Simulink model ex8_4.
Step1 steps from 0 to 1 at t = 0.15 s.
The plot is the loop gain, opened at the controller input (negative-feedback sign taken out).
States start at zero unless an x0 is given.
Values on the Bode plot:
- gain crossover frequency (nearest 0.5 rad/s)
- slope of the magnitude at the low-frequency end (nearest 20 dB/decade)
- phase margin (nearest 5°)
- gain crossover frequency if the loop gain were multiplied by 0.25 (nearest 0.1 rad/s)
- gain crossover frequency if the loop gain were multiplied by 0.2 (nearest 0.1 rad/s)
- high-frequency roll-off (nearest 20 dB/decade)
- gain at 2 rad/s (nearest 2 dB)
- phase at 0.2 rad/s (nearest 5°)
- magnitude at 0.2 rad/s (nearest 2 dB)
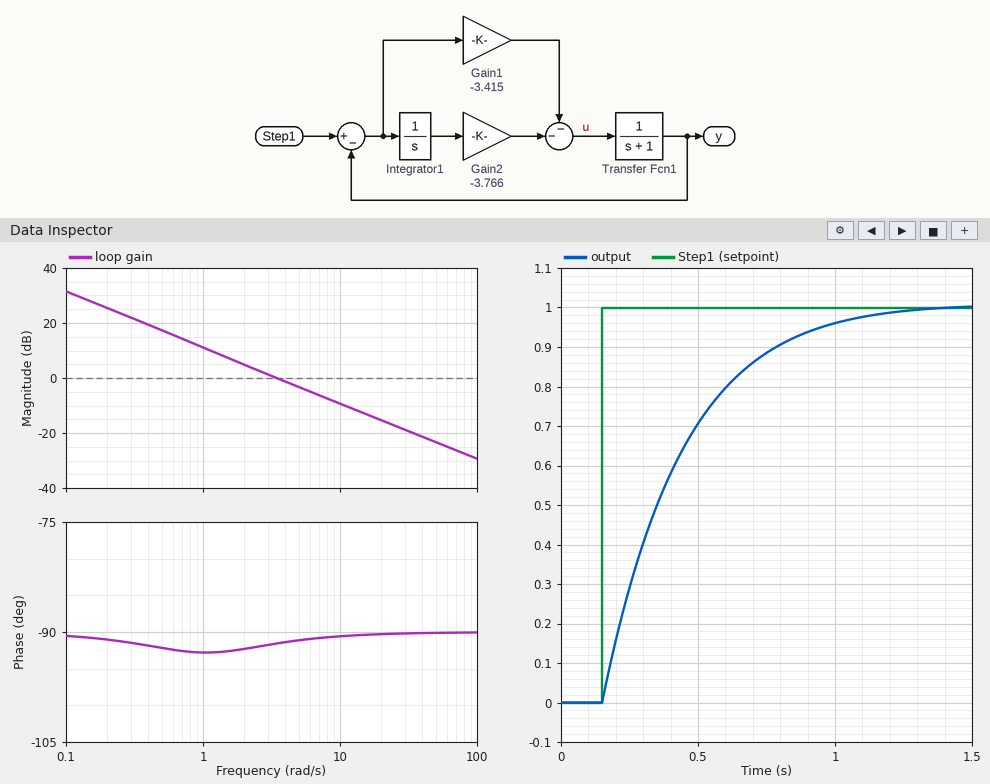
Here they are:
3.5 rad/s
-20 dB/decade
90°
0.9 rad/s
0.7 rad/s
-20 dB/decade
4 dB
-90°
26 dB
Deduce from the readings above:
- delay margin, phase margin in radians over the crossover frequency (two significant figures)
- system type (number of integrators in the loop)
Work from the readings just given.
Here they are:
0.45 s
1
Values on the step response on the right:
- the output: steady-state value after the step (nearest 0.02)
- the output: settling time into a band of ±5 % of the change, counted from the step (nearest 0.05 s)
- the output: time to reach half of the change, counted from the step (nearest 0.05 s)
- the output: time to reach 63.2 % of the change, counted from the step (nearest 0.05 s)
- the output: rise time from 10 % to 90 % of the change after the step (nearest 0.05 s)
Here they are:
1.00
0.80 s
0.20 s
0.30 s
0.60 s
